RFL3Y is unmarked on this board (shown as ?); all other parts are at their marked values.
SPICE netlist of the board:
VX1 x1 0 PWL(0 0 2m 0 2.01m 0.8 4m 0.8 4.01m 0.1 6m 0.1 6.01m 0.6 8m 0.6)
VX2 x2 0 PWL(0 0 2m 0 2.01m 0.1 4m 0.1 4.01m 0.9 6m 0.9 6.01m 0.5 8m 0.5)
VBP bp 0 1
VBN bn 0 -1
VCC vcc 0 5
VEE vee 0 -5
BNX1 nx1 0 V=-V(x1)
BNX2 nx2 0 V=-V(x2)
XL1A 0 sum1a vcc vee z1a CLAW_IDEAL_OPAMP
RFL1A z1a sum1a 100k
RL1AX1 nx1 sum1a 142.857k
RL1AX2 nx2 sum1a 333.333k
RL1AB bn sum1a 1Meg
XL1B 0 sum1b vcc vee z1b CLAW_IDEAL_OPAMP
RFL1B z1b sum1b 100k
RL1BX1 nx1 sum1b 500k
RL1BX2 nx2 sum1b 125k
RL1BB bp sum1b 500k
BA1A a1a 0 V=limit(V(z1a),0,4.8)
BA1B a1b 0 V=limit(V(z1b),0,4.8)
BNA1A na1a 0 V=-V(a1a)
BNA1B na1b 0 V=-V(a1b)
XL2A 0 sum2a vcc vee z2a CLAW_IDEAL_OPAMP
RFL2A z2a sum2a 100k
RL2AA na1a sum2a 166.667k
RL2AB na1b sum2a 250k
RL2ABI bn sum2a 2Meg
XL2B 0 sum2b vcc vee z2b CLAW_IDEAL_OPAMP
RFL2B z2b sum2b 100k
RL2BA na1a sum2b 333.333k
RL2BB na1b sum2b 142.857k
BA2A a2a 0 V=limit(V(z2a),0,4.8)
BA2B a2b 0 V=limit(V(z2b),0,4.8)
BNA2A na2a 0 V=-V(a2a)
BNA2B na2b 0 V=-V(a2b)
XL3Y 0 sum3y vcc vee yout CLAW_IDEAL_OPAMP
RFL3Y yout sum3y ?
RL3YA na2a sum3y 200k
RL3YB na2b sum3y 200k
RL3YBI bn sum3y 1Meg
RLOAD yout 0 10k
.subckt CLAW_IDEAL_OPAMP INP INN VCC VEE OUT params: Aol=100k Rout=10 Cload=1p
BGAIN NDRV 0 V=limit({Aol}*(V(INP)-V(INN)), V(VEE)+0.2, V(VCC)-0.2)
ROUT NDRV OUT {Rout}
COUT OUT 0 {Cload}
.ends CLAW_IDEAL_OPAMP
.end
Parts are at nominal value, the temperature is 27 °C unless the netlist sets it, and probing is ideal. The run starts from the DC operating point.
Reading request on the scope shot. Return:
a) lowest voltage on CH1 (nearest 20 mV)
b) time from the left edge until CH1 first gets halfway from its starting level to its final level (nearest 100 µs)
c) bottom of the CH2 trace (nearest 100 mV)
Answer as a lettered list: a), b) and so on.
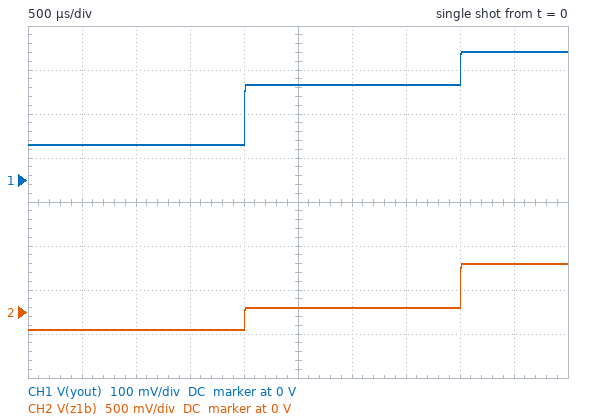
a) 80 mV
b) 2.0 ms
c) -200 mV
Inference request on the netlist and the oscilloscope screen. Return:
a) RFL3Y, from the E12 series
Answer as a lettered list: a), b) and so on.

a) 47 kΩ
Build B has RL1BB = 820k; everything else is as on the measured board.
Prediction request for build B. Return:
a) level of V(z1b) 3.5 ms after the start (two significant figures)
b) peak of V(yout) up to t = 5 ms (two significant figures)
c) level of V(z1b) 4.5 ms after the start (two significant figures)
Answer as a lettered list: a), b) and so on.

a) 120 mV
b) 310 mV
c) 620 mV
